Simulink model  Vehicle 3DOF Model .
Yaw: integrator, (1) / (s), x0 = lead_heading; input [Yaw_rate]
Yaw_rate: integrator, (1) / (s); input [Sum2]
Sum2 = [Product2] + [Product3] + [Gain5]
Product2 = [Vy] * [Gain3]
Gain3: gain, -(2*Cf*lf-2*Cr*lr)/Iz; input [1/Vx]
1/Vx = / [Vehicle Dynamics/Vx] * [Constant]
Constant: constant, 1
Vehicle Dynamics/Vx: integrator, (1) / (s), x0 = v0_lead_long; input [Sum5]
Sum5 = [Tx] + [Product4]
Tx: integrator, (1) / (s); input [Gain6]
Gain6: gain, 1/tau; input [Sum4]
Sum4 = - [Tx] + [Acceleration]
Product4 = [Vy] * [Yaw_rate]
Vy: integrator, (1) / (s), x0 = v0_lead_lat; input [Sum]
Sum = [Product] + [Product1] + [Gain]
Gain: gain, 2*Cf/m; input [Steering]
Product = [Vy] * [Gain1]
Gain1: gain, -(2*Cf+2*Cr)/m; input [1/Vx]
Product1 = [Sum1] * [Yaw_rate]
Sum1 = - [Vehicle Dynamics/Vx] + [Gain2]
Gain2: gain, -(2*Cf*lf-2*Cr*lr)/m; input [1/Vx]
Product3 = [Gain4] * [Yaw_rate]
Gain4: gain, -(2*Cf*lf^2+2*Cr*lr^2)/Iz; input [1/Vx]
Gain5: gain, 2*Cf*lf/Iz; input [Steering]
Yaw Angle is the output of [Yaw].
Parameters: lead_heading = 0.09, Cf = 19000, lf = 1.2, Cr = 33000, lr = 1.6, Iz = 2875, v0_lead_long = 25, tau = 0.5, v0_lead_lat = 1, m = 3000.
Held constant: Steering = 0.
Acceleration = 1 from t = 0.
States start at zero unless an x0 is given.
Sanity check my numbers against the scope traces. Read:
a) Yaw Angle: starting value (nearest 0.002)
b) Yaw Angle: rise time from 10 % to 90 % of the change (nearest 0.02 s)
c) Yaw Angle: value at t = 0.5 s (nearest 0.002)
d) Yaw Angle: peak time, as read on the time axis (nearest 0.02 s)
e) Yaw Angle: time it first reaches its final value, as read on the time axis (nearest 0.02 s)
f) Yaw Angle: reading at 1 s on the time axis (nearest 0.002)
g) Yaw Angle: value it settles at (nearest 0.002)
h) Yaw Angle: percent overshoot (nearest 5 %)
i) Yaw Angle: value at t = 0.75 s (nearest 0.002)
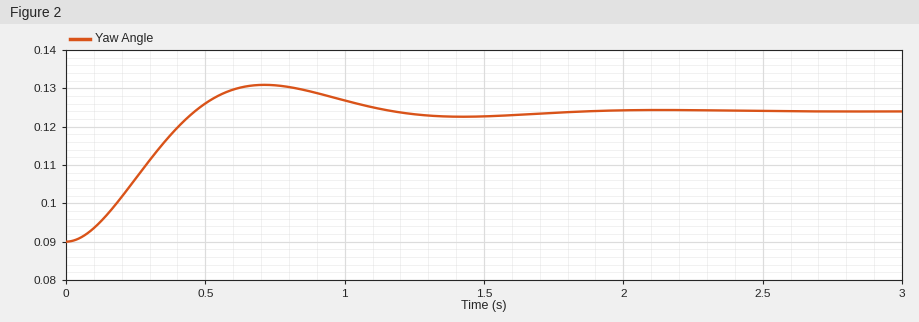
0.090
0.32 s
0.126
0.72 s
0.46 s
0.126
0.124
20 %
0.130
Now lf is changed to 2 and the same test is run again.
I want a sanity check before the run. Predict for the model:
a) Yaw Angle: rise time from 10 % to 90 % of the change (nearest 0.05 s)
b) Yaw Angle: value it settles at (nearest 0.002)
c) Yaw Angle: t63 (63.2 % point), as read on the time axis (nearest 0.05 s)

0.55 s
0.116
0.45 s
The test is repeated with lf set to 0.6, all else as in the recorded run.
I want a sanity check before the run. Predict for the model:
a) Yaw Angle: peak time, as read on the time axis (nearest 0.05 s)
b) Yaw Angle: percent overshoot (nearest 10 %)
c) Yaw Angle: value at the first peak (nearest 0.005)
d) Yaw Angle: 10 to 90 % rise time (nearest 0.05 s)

0.60 s
30 %
0.140
0.25 s
